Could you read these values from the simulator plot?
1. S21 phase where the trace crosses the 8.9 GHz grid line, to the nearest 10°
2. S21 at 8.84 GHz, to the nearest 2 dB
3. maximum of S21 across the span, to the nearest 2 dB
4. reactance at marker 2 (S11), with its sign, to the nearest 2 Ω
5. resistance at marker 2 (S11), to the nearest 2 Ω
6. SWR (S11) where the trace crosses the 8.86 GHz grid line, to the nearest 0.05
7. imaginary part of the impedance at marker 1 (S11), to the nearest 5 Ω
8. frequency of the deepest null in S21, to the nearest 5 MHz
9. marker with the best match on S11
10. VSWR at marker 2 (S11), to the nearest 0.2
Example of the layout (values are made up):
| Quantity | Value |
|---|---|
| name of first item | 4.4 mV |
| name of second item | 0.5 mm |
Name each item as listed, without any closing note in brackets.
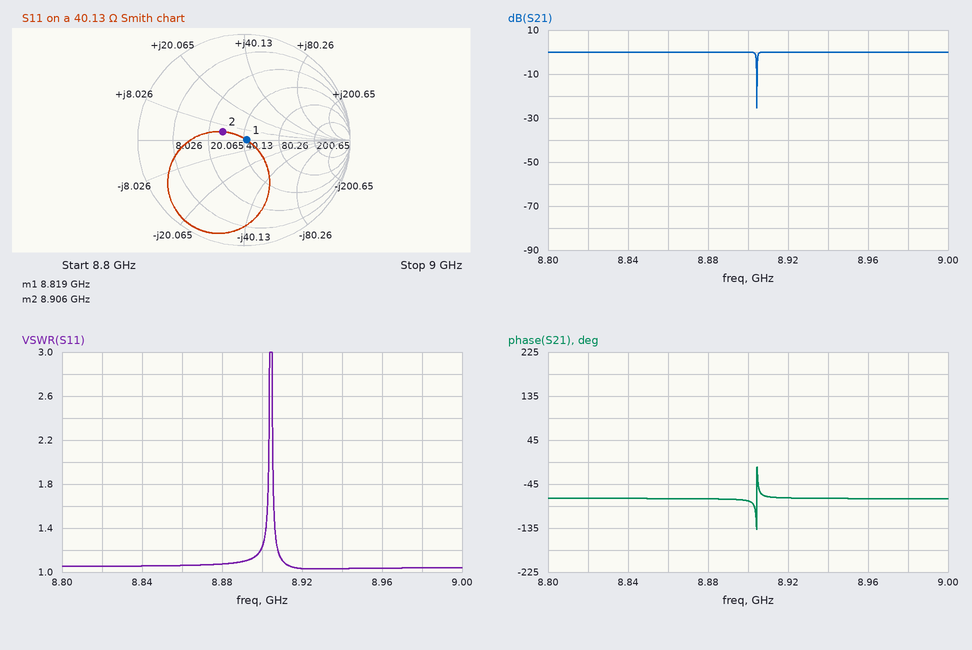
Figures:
| Quantity | Value |
|---|---|
| S21 phase where the trace crosses the 8.9 GHz grid line, to the nearest 10° | -80° |
| S21 at 8.84 GHz, to the nearest 2 dB | 0 dB |
| maximum of S21 across the span, to the nearest 2 dB | 0 dB |
| reactance at marker 2 (S11), with its sign, to the nearest 2 Ω | +4 Ω |
| resistance at marker 2 (S11), to the nearest 2 Ω | 26 Ω |
| SWR (S11) where the trace crosses the 8.86 GHz grid line, to the nearest 0.05 | 1.05 |
| imaginary part of the impedance at marker 1 (S11), to the nearest 5 Ω | 0 Ω |
| frequency of the deepest null in S21, to the nearest 5 MHz | 8.905 GHz |
| marker with the best match on S11 | marker 1 |
| VSWR at marker 2 (S11), to the nearest 0.2 | 1.6 |
